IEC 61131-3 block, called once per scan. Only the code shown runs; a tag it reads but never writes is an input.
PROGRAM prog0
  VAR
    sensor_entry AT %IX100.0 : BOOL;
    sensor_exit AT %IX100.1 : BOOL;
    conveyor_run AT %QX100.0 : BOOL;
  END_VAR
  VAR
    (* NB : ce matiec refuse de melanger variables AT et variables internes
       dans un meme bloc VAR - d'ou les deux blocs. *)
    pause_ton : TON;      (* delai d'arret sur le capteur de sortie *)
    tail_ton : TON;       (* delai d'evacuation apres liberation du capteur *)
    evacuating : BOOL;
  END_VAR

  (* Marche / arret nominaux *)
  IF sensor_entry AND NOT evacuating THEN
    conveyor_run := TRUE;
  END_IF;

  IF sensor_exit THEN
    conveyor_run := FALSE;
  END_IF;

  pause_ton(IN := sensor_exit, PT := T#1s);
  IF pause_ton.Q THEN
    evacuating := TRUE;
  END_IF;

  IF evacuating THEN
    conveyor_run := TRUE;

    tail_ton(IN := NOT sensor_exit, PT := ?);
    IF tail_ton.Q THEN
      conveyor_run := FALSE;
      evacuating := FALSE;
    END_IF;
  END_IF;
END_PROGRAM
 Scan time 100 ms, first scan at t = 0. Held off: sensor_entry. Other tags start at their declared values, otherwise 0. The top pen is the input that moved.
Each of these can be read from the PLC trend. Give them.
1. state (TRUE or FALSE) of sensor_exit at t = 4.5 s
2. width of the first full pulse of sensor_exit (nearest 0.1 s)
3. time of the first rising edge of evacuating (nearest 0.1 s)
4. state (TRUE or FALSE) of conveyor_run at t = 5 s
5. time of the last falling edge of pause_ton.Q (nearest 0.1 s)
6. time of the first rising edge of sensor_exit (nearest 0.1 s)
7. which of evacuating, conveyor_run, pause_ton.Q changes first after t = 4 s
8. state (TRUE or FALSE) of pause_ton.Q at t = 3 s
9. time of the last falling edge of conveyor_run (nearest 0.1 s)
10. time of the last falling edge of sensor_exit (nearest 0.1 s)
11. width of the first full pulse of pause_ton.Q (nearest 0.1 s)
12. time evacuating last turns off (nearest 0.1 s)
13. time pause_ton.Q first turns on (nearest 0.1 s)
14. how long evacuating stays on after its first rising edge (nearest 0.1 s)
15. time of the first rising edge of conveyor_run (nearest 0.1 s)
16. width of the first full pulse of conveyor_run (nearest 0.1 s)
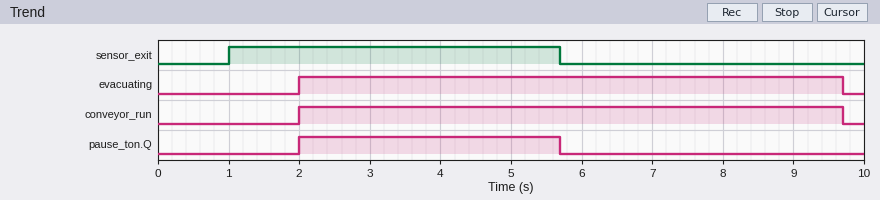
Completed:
TRUE
4.7 s
2.0 s
TRUE
5.7 s
1.0 s
pause_ton.Q
TRUE
9.7 s
5.7 s
3.7 s
9.7 s
2.0 s
7.7 s
2.0 s
7.7 s
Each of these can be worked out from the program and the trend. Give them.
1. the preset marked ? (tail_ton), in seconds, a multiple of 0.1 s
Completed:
4.0 s
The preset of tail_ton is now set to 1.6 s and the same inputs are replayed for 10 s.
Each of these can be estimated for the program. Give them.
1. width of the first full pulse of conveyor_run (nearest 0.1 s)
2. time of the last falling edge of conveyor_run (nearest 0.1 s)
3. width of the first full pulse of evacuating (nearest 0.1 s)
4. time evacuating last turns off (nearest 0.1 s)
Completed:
5.3 s
7.3 s
5.3 s
7.3 s
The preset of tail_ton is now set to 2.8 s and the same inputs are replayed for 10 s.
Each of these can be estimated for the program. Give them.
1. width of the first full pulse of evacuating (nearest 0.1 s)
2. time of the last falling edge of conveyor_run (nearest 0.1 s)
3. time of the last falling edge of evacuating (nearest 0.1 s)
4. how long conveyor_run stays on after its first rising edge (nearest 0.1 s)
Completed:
6.5 s
8.5 s
8.5 s
6.5 s
